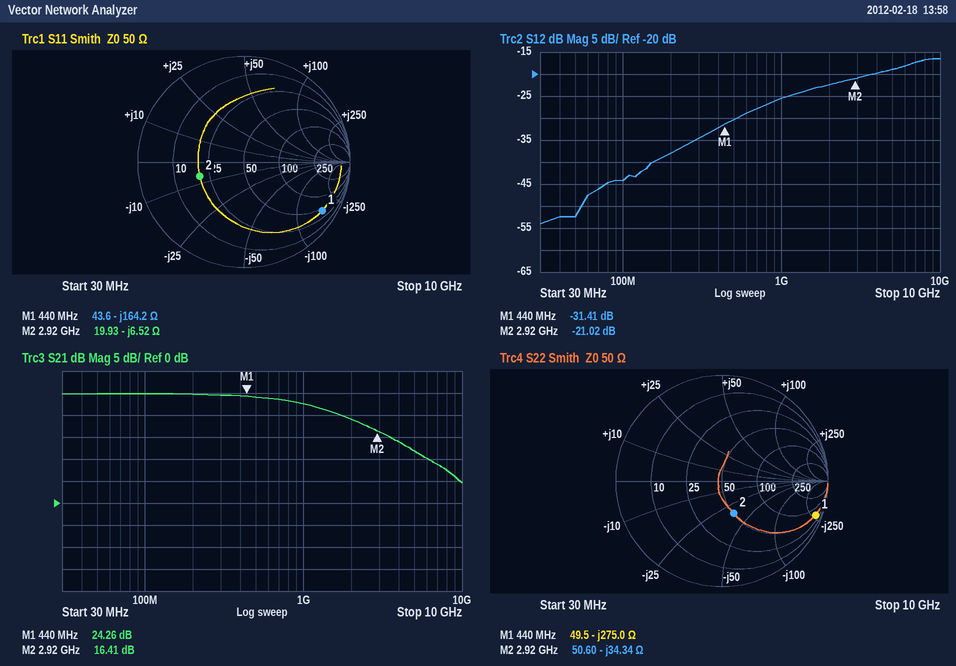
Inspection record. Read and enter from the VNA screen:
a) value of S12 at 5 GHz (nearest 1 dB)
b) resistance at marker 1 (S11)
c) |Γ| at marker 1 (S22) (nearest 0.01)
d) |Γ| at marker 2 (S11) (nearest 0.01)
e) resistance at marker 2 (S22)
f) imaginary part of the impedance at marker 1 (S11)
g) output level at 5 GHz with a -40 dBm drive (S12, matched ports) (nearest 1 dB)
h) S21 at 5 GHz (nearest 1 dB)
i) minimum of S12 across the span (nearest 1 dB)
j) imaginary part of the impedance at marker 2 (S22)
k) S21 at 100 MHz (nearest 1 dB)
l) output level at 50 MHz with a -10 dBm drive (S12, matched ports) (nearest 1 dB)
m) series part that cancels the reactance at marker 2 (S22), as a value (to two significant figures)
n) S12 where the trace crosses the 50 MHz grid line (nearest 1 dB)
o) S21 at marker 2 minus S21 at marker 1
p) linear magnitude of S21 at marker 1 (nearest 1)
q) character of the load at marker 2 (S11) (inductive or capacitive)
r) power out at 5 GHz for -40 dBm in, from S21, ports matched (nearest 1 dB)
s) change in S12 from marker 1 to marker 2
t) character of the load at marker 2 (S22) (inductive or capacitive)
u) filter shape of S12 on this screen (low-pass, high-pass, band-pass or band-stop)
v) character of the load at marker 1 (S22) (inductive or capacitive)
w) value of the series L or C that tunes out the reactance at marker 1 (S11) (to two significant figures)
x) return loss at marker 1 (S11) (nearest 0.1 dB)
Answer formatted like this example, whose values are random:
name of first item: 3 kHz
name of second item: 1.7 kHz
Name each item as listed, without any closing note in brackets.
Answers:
value of S12 at 5 GHz: -19 dB
resistance at marker 1: 43.6 Ω
|Γ| at marker 1 (S22): 0.94
|Γ| at marker 2 (S11): 0.44
resistance at marker 2: 50.60 Ω
imaginary part of the impedance at marker 1: -164.2 Ω
output level at 5 GHz with a -40 dBm drive (S12, matched ports): -59 dBm
S21 at 5 GHz: 12 dB
minimum of S12 across the span: -54 dB
imaginary part of the impedance at marker 2: -34.34 Ω
S21 at 100 MHz: 25 dB
output level at 50 MHz with a -10 dBm drive (S12, matched ports): -62 dBm
series part that cancels the reactance at marker 2 (S22), as a value: 1.9 nH
S12 where the trace crosses the 50 MHz grid line: -52 dB
S21 at marker 2 minus S21 at marker 1: -7.85 dB
linear magnitude of S21 at marker 1: 16
character of the load at marker 2 (S11): capacitive
power out at 5 GHz for -40 dBm in, from S21, ports matched: -28 dBm
change in S12 from marker 1 to marker 2: 10.39 dB
character of the load at marker 2 (S22): capacitive
filter shape of S12 on this screen: high-pass
character of the load at marker 1 (S22): capacitive
value of the series L or C that tunes out the reactance at marker 1 (S11): 59 nH
return loss at marker 1 (S11): 1.2 dB
